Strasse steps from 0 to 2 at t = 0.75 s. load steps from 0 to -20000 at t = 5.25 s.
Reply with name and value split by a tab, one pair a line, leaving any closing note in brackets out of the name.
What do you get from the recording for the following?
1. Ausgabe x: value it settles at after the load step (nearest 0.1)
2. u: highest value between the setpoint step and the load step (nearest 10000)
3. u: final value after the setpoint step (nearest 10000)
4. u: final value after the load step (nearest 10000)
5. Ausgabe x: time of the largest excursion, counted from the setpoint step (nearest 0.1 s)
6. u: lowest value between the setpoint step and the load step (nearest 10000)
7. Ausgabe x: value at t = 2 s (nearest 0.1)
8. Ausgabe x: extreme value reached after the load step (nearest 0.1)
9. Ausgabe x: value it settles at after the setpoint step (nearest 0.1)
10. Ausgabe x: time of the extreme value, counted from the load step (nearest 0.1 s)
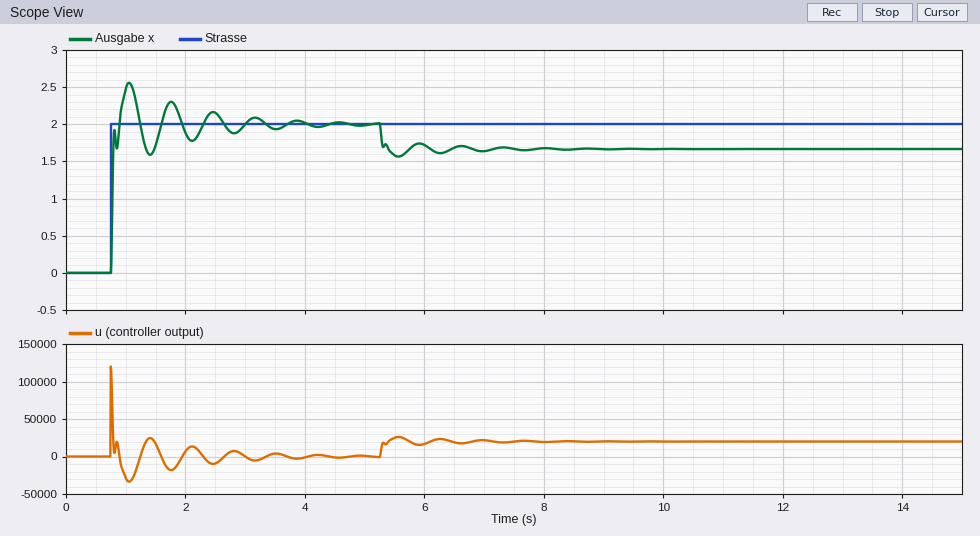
Ausgabe x: value it settles at after the load step	1.7
u: highest value between the setpoint step and the load step	120000
u: final value after the setpoint step	0
u: final value after the load step	20000
Ausgabe x: time of the largest excursion, counted from the setpoint step	0.3 s
u: lowest value between the setpoint step and the load step	-30000
Ausgabe x: value at t = 2 s	1.9
Ausgabe x: extreme value reached after the load step	1.6
Ausgabe x: value it settles at after the setpoint step	2.0
Ausgabe x: time of the extreme value, counted from the load step	0.3 s
